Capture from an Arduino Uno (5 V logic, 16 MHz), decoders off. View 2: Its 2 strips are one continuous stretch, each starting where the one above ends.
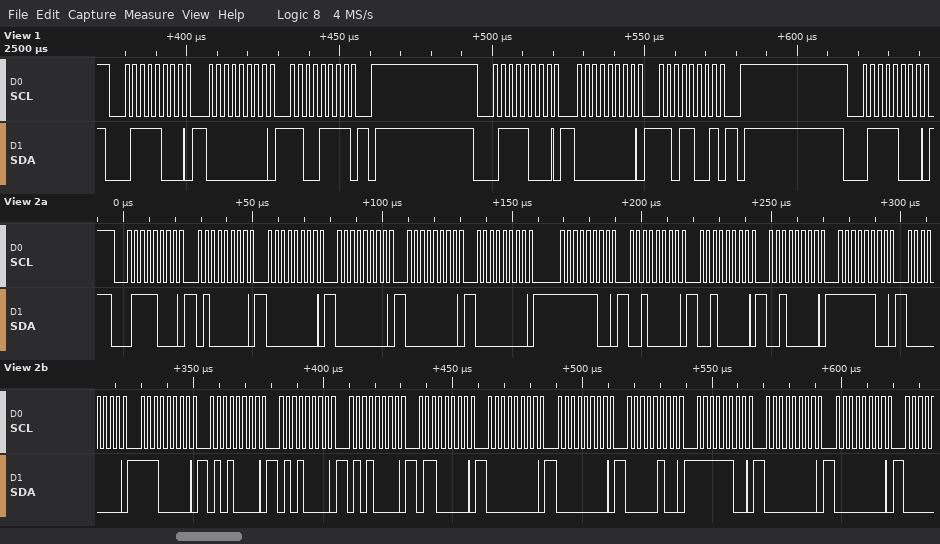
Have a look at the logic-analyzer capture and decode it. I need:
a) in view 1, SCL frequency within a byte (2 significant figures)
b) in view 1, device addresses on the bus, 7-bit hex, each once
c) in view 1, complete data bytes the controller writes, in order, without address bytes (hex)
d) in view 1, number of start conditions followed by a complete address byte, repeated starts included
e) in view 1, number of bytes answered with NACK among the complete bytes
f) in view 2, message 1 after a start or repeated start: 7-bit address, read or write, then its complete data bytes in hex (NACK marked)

400 kHz
0x3C
00 CF 00 D9
3
0
0x3C write: 40 00 00 00 00 FC 20 20 20 FC 00 E0 50 50 50 60 00 00 04 FC 00 00
